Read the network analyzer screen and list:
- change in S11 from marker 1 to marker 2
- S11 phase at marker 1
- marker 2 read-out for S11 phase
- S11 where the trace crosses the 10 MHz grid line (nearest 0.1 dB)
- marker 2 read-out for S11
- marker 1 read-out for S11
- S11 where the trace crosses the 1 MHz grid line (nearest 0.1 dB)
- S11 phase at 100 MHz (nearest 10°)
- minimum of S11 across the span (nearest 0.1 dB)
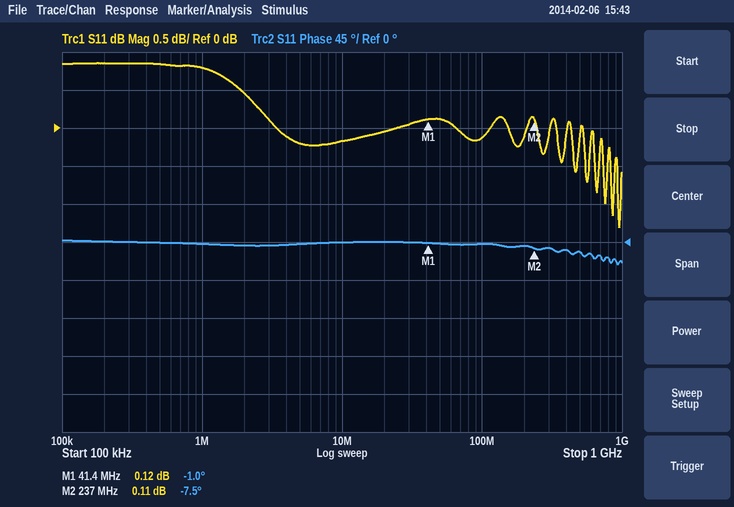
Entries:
-0.01 dB
-1.0°
-7.5°
-0.2 dB
0.11 dB
0.12 dB
0.8 dB
0°
-1.3 dB
